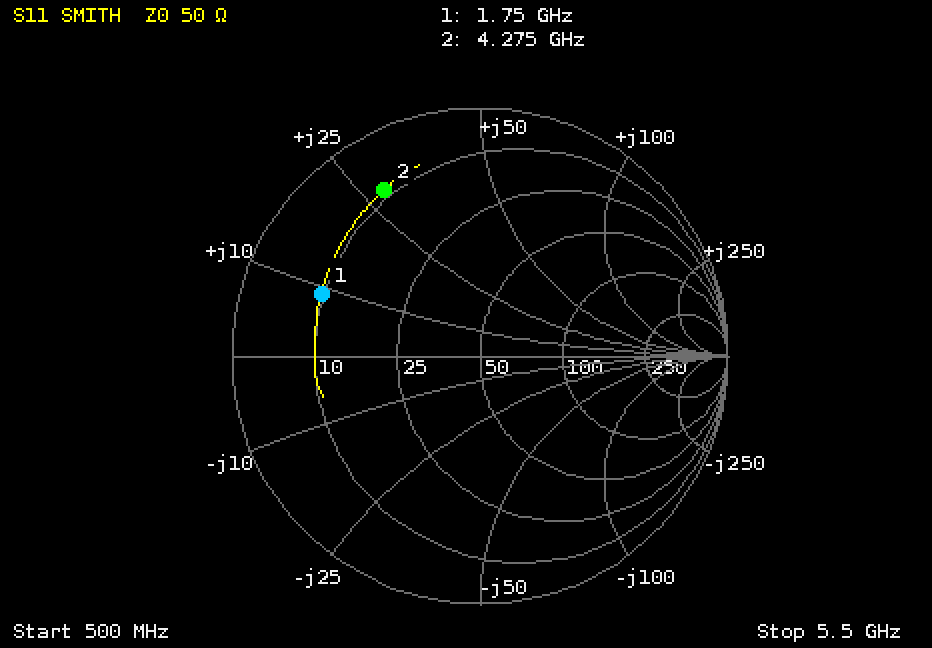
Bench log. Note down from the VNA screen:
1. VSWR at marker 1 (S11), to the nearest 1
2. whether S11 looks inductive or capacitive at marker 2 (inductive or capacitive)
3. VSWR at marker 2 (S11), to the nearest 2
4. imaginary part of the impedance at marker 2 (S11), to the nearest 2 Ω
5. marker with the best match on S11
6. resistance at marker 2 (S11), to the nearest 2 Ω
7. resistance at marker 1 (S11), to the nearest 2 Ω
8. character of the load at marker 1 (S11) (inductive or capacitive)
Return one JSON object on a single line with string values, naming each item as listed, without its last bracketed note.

{"VSWR at marker 1 (S11), to the nearest 1": "5", "whether S11 looks inductive or capacitive at marker 2": "inductive", "VSWR at marker 2 (S11), to the nearest 2": "8", "imaginary part of the impedance at marker 2 (S11), to the nearest 2 Ω": "+28 Ω", "marker with the best match on S11": "marker 1", "resistance at marker 2 (S11), to the nearest 2 Ω": "8 Ω", "resistance at marker 1 (S11), to the nearest 2 Ω": "10 Ω", "character of the load at marker 1 (S11)": "inductive"}
